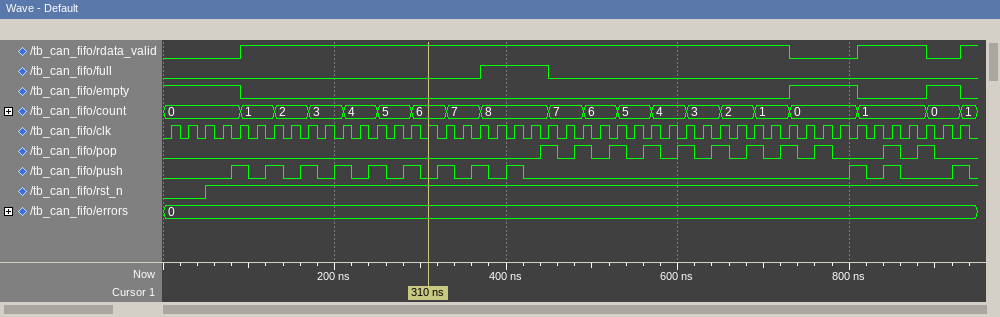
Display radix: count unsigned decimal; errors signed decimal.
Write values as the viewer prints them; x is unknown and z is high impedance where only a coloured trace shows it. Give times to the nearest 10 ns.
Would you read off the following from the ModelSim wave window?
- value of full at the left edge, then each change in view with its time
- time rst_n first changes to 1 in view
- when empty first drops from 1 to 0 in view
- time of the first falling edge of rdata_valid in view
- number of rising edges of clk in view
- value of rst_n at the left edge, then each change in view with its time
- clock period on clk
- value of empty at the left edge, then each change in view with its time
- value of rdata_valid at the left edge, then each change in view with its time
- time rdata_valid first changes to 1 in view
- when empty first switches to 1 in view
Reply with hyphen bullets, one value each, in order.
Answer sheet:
- 0, 1 at 370 ns, 0 at 450 ns
- 50 ns
- 90 ns
- 730 ns
- 47
- 0, 1 at 50 ns
- 20 ns
- 1, 0 at 90 ns, 1 at 730 ns, 0 at 810 ns, 1 at 890 ns, 0 at 930 ns
- 0, 1 at 90 ns, 0 at 730 ns, 1 at 810 ns, 0 at 890 ns, 1 at 930 ns
- 90 ns
- 730 ns
